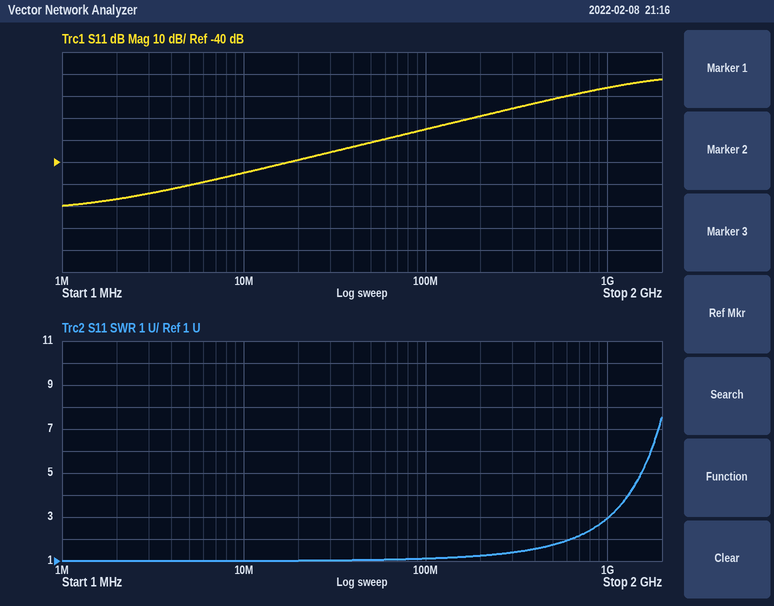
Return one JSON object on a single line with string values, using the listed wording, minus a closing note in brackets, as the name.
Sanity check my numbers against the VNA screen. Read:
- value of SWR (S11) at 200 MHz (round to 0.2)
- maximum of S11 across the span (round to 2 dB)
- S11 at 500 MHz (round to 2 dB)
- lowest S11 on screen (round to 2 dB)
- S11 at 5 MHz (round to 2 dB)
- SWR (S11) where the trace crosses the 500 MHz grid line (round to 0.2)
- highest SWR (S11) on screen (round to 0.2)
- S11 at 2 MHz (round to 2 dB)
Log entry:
{"value of SWR (S11) at 200 MHz": "1.2", "maximum of S11 across the span": "-2 dB", "S11 at 500 MHz": "-12 dB", "lowest S11 on screen": "-60 dB", "S11 at 5 MHz": "-50 dB", "SWR (S11) where the trace crosses the 500 MHz grid line": "1.8", "highest SWR (S11) on screen": "7.6", "S11 at 2 MHz": "-56 dB"}
